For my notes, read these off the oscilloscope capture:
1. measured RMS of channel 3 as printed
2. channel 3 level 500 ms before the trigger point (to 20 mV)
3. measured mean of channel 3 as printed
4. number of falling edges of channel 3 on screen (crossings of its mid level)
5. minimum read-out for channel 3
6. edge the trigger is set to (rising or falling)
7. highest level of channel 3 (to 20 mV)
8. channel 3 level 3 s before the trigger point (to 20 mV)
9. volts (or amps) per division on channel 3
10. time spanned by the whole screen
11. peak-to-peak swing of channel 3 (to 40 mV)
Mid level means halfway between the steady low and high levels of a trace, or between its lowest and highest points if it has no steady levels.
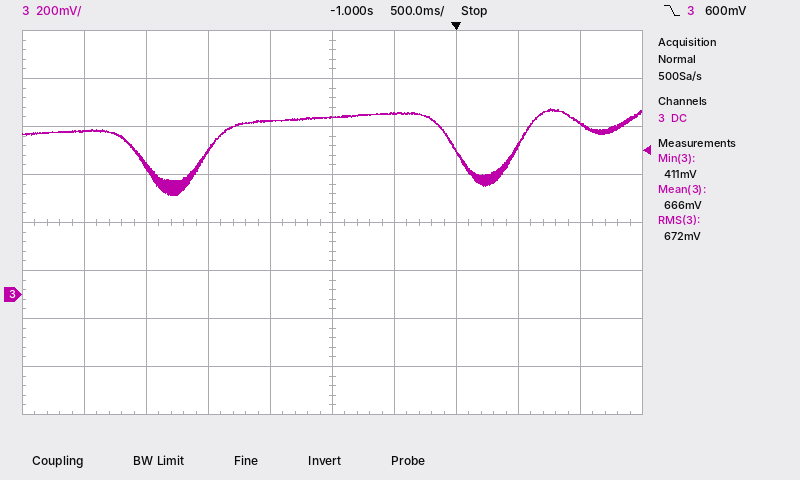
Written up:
672 mV
760 mV
666 mV
2
411 mV
falling
780 mV
680 mV
200 mV
5 s
360 mV
